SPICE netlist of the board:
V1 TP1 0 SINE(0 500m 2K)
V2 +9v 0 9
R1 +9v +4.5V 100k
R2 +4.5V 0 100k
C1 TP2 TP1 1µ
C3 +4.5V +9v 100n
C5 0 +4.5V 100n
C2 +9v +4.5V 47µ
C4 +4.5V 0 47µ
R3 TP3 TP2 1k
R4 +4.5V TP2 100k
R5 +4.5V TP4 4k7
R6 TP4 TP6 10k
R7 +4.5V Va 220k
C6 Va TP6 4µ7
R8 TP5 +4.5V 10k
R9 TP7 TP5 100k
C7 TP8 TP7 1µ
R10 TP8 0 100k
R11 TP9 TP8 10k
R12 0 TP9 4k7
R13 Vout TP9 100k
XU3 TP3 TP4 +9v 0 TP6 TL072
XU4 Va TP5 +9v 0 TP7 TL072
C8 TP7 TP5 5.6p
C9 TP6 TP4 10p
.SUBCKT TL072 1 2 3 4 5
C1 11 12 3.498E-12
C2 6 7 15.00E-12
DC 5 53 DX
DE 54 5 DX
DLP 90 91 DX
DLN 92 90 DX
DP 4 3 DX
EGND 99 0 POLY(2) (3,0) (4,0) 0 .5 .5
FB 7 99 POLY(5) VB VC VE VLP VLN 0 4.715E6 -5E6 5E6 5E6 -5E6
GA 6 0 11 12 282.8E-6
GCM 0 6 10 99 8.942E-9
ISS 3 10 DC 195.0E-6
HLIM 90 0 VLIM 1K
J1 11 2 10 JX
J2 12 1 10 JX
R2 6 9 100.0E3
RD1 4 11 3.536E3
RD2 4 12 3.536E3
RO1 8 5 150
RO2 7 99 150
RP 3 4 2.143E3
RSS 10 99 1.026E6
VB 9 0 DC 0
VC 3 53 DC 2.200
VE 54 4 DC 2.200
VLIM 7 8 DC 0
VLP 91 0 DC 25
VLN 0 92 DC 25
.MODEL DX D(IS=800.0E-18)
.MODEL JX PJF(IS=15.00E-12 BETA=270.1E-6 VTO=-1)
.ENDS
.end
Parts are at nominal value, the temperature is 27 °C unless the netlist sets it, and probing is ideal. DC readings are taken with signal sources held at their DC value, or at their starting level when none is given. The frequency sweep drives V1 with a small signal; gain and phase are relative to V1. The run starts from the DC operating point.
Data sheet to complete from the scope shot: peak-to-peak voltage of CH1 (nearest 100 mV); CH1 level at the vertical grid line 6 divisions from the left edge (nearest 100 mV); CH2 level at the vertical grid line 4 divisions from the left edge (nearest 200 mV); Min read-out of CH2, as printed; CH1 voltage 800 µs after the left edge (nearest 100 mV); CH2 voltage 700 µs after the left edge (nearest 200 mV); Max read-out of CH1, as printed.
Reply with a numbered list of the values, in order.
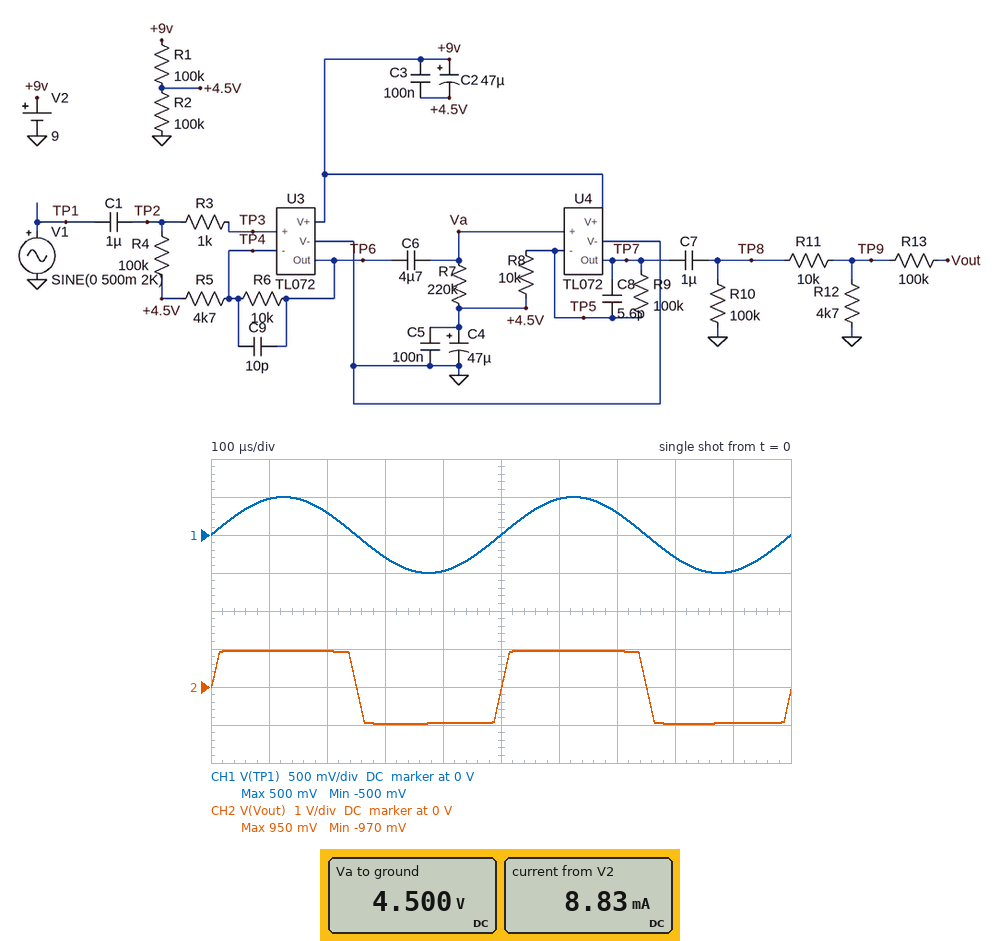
1. 1.0 V
2. 500 mV
3. -1.0 V
4. -970 mV
5. -300 mV
6. 1.0 V
7. 500 mV
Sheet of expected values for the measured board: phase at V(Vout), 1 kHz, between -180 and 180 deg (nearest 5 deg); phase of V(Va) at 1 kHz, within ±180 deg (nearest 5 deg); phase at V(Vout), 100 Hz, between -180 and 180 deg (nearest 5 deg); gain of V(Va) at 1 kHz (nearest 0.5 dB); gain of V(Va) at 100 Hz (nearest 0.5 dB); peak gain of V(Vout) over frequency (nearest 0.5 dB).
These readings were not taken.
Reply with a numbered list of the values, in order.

1. 0 deg
2. 0 deg
3. 10 deg
4. 10.0 dB
5. 10.0 dB
6. 21.0 dB
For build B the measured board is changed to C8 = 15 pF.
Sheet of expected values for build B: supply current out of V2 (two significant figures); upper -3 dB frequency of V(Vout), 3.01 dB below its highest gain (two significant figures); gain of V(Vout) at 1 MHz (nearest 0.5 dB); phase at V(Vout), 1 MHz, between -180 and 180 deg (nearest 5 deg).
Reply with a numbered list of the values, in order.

1. 8.8 mA
2. 80 kHz
3. -3.0 dB
4. -115 deg
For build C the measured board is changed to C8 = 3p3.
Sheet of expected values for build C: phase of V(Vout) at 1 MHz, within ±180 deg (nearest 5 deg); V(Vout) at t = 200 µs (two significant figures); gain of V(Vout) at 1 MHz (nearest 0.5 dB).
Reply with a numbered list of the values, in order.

1. -135 deg
2. 940 mV
3. 2.5 dB
